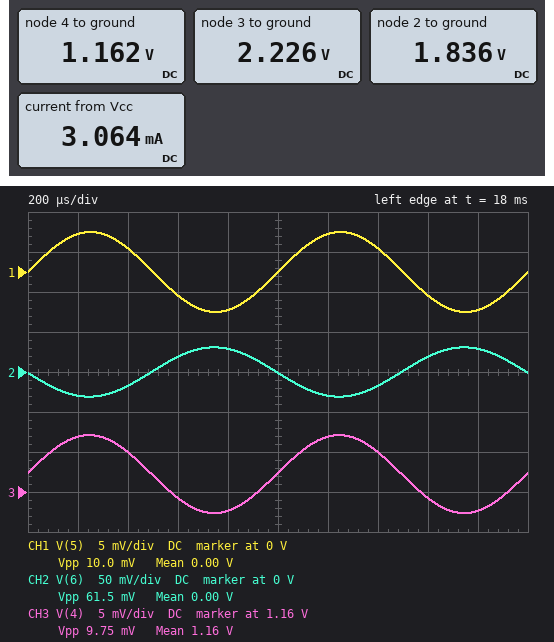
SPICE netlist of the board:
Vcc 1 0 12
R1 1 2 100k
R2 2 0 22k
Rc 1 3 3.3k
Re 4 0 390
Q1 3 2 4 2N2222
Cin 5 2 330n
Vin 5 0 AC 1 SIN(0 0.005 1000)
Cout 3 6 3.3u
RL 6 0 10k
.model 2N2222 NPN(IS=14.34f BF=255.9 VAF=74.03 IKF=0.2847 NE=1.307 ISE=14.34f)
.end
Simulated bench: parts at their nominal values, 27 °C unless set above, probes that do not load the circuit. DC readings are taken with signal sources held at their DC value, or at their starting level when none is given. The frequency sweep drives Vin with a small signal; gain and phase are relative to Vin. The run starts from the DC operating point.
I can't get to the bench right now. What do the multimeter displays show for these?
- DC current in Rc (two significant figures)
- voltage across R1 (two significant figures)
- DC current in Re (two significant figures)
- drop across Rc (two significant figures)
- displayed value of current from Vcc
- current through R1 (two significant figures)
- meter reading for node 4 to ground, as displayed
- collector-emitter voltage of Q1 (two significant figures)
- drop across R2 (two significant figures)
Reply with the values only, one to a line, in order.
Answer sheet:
3.0 mA
10 V
3.0 mA
9.8 V
3.064 mA
100 µA
1.162 V
1.1 V
1.8 V
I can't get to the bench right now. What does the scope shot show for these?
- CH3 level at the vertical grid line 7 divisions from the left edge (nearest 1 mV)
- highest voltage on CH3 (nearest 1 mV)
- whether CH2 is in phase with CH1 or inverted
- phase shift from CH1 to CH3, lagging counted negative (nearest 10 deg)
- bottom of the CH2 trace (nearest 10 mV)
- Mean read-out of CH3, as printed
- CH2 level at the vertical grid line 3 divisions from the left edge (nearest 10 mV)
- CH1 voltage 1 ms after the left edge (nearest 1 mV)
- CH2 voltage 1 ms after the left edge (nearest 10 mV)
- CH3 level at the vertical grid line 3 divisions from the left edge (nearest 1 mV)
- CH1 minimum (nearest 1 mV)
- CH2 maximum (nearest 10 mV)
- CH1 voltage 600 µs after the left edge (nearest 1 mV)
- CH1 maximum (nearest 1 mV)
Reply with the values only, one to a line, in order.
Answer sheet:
1.165 V
1.167 V
inverted
0 deg
-30 mV
1.16 V
20 mV
0 V
0 V
1.159 V
-5 mV
30 mV
-3 mV
5 mV
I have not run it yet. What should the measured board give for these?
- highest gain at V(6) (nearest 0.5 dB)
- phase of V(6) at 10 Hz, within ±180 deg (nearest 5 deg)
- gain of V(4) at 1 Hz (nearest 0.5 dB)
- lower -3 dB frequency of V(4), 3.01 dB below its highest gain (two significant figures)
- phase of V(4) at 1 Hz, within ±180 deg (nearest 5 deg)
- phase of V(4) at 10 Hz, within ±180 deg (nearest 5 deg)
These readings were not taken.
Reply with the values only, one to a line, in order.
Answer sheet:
16.0 dB
-85 deg
-31.0 dB
34 Hz
90 deg
75 deg
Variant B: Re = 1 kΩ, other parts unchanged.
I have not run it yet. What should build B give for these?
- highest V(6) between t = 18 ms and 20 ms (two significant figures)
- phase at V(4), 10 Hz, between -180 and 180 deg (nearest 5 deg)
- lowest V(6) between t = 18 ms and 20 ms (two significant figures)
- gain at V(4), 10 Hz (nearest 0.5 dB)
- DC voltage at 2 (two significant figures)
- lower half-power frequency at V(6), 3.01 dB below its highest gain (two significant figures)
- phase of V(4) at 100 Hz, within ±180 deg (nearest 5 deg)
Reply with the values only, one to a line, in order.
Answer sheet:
12 mV
70 deg
-12 mV
-10.0 dB
2.0 V
30 Hz
15 deg
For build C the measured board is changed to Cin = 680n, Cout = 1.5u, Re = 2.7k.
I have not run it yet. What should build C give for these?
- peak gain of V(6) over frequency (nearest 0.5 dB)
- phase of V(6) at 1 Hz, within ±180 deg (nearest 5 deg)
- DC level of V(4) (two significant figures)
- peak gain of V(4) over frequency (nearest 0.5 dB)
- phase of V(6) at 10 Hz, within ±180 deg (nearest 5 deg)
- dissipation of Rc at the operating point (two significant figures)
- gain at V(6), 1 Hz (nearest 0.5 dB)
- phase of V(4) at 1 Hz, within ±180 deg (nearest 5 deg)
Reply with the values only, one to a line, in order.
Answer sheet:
-1.0 dB
-10 deg
1.5 V
0 dB
-90 deg
970 µW
-41.5 dB
85 deg
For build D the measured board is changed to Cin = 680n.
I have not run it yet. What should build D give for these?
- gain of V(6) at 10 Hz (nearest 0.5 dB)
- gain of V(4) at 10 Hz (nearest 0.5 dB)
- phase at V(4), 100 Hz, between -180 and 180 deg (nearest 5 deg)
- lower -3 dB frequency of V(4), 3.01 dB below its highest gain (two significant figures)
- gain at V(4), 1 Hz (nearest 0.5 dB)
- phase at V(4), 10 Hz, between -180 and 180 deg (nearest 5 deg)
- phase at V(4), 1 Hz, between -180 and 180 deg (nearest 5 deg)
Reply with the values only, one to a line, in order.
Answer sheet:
9.5 dB
-6.0 dB
10 deg
17 Hz
-24.5 dB
60 deg
85 deg
